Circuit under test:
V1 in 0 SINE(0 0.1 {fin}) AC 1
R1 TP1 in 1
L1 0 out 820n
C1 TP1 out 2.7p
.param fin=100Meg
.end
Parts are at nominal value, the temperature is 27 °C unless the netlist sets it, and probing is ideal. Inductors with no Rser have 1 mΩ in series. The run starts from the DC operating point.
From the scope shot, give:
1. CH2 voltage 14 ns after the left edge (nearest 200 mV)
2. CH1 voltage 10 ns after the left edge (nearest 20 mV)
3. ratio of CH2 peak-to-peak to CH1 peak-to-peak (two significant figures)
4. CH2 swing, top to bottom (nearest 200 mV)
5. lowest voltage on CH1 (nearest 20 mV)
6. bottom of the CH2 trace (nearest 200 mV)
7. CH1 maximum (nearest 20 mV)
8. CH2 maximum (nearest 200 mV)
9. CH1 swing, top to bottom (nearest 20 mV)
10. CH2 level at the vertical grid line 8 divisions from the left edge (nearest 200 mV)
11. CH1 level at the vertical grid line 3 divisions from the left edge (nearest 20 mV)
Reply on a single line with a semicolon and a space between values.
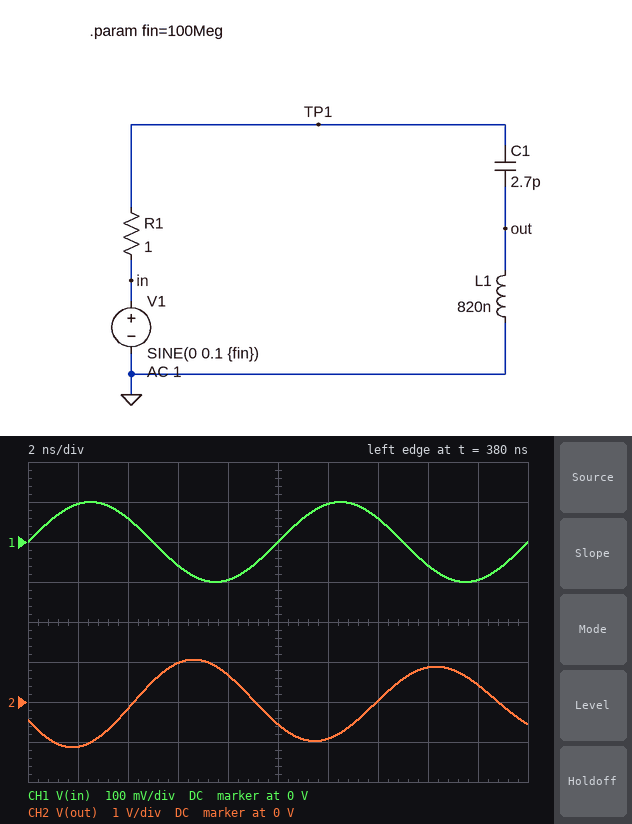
0 V; 0 V; 11; 2.2 V; -100 mV; -1.2 V; 100 mV; 1.0 V; 200 mV; 800 mV; -60 mV
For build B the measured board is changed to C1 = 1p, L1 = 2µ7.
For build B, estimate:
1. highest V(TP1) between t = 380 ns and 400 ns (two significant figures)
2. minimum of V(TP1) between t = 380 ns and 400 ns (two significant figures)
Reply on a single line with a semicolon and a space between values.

99 mV; -99 mV
